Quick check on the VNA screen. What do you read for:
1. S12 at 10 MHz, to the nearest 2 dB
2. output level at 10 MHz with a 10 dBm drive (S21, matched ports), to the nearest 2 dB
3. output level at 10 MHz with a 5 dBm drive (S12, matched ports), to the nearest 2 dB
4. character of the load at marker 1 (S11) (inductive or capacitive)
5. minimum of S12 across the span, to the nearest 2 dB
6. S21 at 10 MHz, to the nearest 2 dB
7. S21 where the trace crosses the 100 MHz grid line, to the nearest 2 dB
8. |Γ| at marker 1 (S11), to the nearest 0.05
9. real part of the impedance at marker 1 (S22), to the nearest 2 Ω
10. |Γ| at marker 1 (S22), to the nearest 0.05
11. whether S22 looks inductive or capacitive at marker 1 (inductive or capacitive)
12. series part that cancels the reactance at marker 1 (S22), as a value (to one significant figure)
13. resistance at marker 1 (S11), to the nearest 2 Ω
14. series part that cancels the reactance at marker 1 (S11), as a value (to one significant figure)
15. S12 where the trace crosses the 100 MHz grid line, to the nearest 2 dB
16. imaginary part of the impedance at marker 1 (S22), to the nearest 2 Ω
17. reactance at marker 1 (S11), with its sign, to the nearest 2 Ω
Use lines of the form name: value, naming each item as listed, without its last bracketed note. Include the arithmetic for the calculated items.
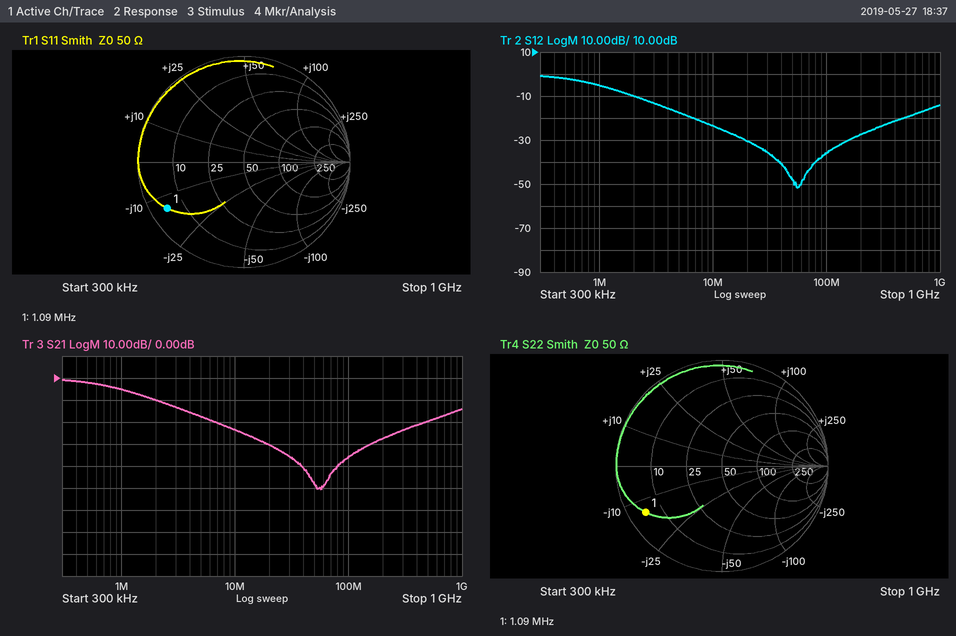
S12 at 10 MHz, to the nearest 2 dB: -24 dB
output level at 10 MHz with a 10 dBm drive (S21, matched ports), to the nearest 2 dB: 10 dBm + (-24 dB) = -14 dBm
output level at 10 MHz with a 5 dBm drive (S12, matched ports), to the nearest 2 dB: 5 dBm + (-24 dB) = -18 dBm
character of the load at marker 1 (S11): capacitive
minimum of S12 across the span, to the nearest 2 dB: -52 dB
S21 at 10 MHz, to the nearest 2 dB: -24 dB
S21 where the trace crosses the 100 MHz grid line, to the nearest 2 dB: -36 dB
|Γ| at marker 1 (S11), to the nearest 0.05: 0.85
real part of the impedance at marker 1 (S22), to the nearest 2 Ω: 4 Ω
|Γ| at marker 1 (S22), to the nearest 0.05: 0.85
whether S22 looks inductive or capacitive at marker 1: capacitive
series part that cancels the reactance at marker 1 (S22), as a value: L = 14 Ω/(2π × 1.09 MHz) ≈ 2 µH
resistance at marker 1 (S11), to the nearest 2 Ω: 4 Ω
series part that cancels the reactance at marker 1 (S11), as a value: L = 14 Ω/(2π × 1.09 MHz) ≈ 2 µH
S12 where the trace crosses the 100 MHz grid line, to the nearest 2 dB: -36 dB
imaginary part of the impedance at marker 1 (S22), to the nearest 2 Ω: -14 Ω
reactance at marker 1 (S11), with its sign, to the nearest 2 Ω: -14 Ω
